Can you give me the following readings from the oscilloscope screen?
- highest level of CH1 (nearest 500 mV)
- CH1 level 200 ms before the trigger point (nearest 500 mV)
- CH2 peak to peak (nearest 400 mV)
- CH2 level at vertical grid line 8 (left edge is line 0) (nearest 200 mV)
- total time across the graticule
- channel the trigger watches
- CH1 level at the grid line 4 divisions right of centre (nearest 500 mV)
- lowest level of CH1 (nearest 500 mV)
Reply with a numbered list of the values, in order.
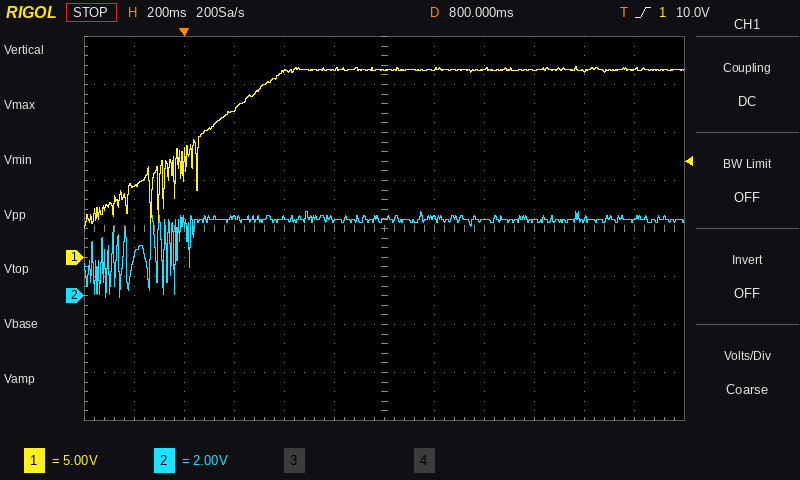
1. 20.0 V
2. 7.5 V
3. 3.6 V
4. 3.2 V
5. 2.4 s
6. CH1
7. 19.5 V
8. 3.0 V
